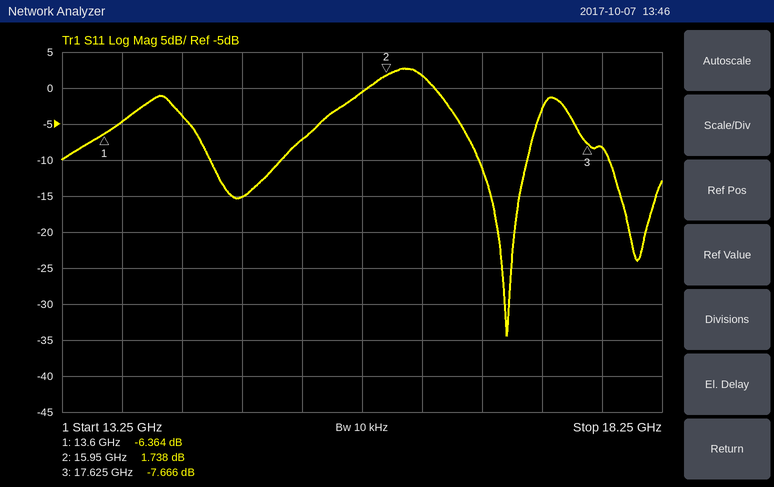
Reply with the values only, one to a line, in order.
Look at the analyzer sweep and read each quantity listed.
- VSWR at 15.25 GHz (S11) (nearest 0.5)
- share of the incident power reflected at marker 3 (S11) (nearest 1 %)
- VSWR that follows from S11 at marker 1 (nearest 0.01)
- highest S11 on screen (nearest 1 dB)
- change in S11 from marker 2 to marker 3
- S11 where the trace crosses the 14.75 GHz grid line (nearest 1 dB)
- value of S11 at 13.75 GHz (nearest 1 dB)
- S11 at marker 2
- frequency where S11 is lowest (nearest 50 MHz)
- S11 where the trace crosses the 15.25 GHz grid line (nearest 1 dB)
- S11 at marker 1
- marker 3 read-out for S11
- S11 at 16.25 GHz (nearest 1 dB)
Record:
2.5
17 %
2.85
3 dB
-9.404 dB
-15 dB
-5 dB
1.738 dB
16.95 GHz
-7 dB
-6.364 dB
-7.666 dB
2 dB
